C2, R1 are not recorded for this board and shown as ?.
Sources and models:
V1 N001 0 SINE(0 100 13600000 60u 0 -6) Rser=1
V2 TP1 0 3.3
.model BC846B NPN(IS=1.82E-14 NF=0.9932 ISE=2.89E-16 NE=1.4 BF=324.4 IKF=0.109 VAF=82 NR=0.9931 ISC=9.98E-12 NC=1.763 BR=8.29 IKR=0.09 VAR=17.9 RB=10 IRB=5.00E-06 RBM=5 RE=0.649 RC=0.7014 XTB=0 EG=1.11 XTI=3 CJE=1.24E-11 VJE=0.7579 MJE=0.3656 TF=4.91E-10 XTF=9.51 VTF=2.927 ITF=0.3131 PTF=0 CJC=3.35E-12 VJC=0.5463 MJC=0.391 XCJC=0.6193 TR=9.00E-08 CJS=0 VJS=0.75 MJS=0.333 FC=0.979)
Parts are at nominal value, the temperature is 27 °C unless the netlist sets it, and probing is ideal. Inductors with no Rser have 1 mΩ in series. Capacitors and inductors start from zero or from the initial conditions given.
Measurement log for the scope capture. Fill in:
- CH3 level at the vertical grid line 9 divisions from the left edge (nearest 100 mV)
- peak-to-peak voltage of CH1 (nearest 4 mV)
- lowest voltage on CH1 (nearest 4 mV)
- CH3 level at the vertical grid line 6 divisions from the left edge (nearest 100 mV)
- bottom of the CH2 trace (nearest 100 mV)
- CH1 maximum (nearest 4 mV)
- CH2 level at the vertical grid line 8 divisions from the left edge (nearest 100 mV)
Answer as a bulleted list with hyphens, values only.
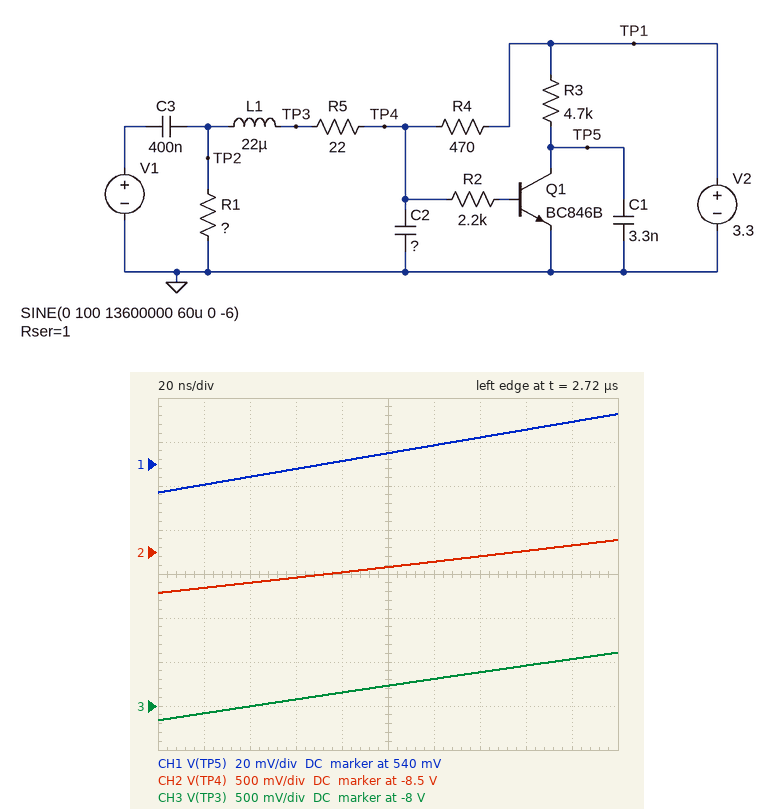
- -7.5 V
- 36 mV
- 528 mV
- -7.7 V
- -9.0 V
- 564 mV
- -8.5 V
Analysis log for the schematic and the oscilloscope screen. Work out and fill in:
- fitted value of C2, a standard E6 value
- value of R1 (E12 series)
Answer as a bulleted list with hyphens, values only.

- 22 nF
- 22 Ω
